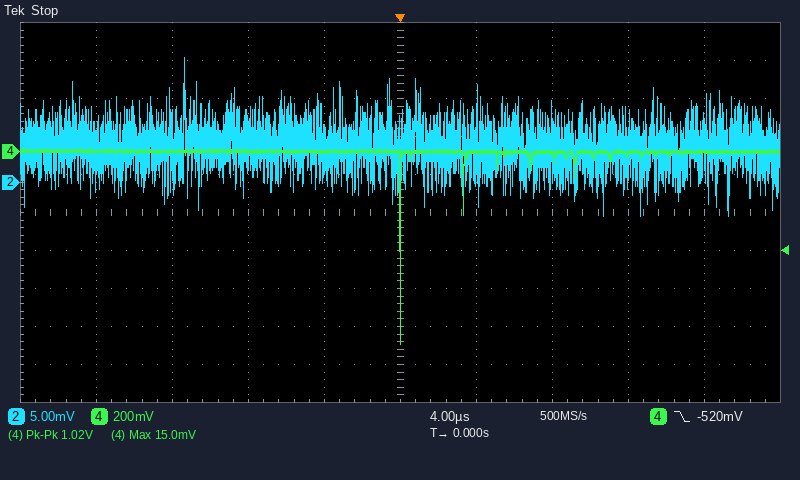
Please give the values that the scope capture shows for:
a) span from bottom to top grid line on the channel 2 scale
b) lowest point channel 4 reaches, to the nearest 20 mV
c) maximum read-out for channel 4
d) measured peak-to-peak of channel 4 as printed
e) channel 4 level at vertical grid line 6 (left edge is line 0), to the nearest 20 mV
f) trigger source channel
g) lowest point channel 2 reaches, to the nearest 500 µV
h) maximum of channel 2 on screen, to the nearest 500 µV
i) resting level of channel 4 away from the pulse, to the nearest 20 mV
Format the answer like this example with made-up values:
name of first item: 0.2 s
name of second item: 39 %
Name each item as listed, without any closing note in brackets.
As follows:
span from bottom to top grid line on the channel 2 scale: 50 mV
lowest point channel 4 reaches, to the nearest 20 mV: -1.00 V
maximum read-out for channel 4: 15.0 mV
measured peak-to-peak of channel 4 as printed: 1.02 V
channel 4 level at vertical grid line 6 (left edge is line 0), to the nearest 20 mV: 0 mV
trigger source channel: channel 4
lowest point channel 2 reaches, to the nearest 500 µV: -4.5 mV
maximum of channel 2 on screen, to the nearest 500 µV: 16.5 mV
resting level of channel 4 away from the pulse, to the nearest 20 mV: 0 mV
